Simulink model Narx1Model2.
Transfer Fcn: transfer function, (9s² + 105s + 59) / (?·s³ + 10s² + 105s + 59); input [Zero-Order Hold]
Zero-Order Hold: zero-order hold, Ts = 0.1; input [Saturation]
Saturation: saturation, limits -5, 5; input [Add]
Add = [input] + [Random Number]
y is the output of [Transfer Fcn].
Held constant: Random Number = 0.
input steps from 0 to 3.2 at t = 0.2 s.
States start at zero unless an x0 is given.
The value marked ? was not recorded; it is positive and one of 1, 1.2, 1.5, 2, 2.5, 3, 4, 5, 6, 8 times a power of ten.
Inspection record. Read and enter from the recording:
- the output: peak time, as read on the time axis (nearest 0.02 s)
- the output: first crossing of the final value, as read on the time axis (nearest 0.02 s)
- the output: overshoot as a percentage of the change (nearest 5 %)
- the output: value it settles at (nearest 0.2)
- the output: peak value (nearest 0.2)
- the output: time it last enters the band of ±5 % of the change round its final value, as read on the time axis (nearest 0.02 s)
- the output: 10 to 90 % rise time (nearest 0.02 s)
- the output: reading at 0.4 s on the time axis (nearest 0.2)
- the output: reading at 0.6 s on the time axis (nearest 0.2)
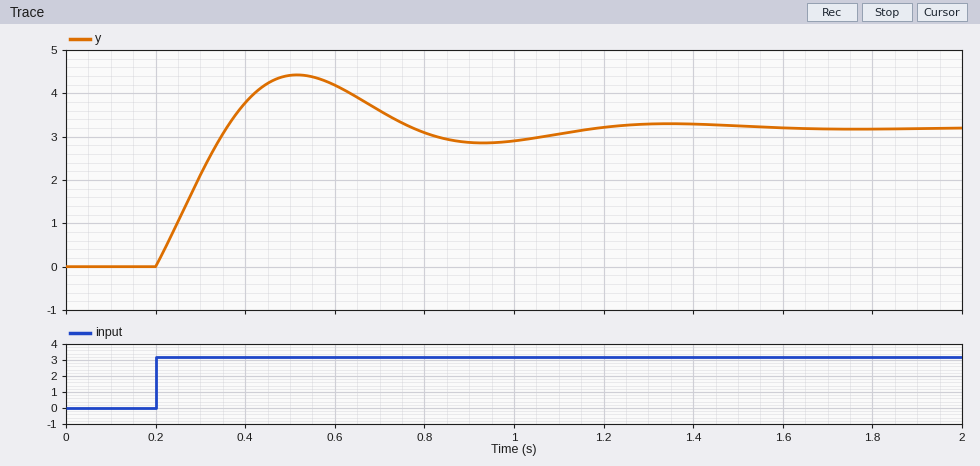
0.52 s
0.36 s
40 %
3.2
4.4
1.08 s
0.12 s
3.8
4.2
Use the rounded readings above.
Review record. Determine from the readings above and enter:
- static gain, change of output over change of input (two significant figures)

1.0
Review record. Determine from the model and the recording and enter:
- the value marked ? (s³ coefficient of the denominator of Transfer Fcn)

1.5
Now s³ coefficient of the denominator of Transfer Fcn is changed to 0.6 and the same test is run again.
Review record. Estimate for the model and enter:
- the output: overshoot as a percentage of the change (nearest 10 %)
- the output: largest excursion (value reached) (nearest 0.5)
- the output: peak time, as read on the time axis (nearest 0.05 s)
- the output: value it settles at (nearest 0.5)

20 %
4.0
0.40 s
3.0
